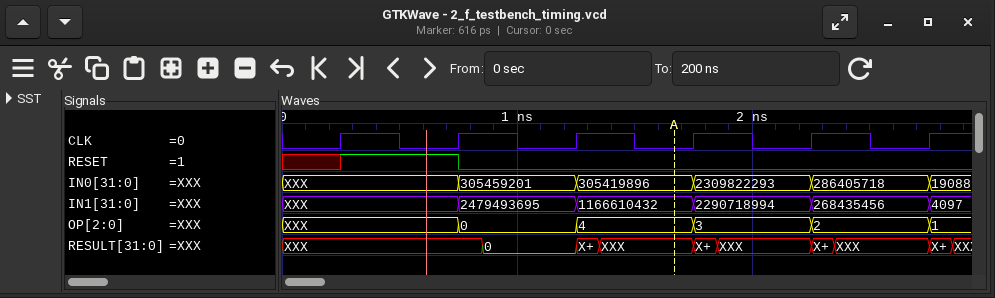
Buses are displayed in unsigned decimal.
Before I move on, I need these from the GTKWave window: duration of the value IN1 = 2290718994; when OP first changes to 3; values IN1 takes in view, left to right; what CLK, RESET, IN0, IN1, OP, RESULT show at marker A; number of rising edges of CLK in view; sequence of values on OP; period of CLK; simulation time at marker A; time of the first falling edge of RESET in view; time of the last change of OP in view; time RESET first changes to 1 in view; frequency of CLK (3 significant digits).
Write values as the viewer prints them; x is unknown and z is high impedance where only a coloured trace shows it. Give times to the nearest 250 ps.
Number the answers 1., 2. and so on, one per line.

1. 500 ps
2. 1750 ps
3. XXX, 2479493695, 1166610432, 2290718994, 268435456, 4097
4. CLK=0, RESET=0, IN0=305419896, IN1=1166610432, OP=4, RESULT=XXX
5. 6
6. XXX, 0, 4, 3, 2, 1
7. 500 ps
8. 1750 ps
9. 750 ps
10. 2750 ps
11. 250 ps
12. 2.00 GHz
